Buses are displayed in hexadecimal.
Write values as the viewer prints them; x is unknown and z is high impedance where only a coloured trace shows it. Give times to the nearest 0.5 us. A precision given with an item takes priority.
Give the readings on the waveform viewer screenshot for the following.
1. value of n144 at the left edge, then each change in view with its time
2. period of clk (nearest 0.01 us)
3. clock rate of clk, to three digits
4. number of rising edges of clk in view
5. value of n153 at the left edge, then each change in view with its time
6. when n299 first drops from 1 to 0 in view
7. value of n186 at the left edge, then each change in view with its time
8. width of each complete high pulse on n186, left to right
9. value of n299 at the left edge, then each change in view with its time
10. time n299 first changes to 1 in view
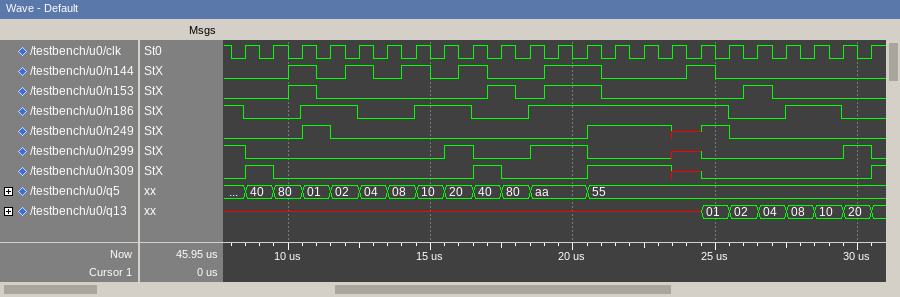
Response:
0, 1 at 10 us, 0 at 11 us, 1 at 12 us, 0 at 13 us, 1 at 14 us, 0 at 15 us, 1 at 16 us, 0 at 17 us, 1 at 19 us, 0 at 21 us, 1 at 24 us, 0 at 25 us
1 us
1.00 MHz
23
0, 1 at 10 us, 0 at 11 us, 1 at 17 us, 0 at 18 us, 1 at 19 us, 0 at 21 us, 1 at 26 us, 0 at 27 us
8.5 us
1, 0 at 8.5 us, 1 at 10.5 us, 0 at 12.5 us, 1 at 14.5 us, 0 at 16.5 us, 1 at 18.5 us, 0 at 25.5 us, 1 at 27.5 us, 0 at 29.5 us
2 us, 2 us, 7 us, 2 us
1, 0 at 8.5 us, 1 at 15.5 us, 0 at 16.5 us, 1 at 18.5 us, 0 at 20.5 us, x at 23.5 us, 0 at 24.5 us, 1 at 29.5 us, 0 at 30.5 us
15.5 us
